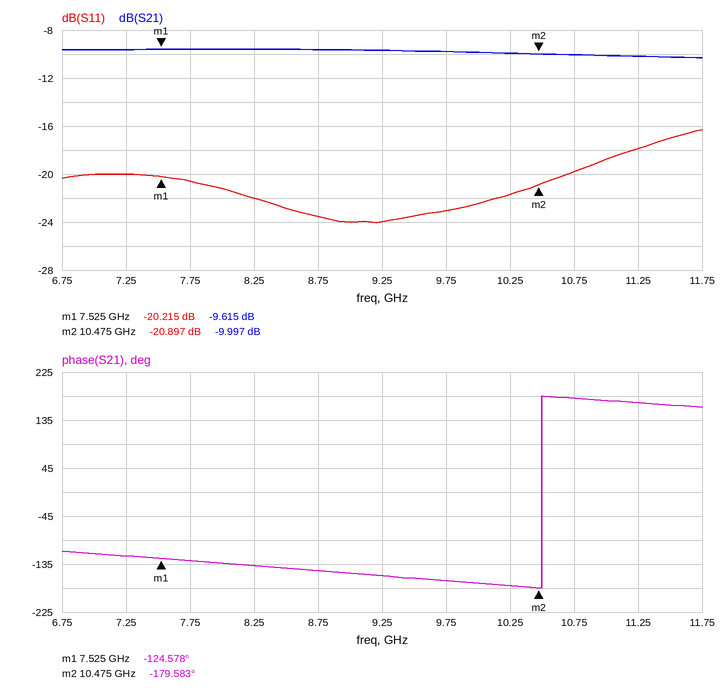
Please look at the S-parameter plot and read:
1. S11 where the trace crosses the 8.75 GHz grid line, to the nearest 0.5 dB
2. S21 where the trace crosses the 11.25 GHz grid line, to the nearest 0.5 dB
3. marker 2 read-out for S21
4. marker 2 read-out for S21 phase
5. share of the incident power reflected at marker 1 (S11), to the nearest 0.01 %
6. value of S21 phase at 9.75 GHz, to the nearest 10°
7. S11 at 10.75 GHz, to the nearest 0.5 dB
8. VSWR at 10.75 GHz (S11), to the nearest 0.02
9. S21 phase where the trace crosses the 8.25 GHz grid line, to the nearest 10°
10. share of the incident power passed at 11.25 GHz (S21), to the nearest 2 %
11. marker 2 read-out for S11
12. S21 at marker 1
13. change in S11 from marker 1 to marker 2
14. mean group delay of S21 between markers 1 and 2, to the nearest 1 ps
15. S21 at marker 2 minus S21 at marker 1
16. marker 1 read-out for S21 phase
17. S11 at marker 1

-23.5 dB
-10.0 dB
-9.997 dB
-179.583°
0.95 %
-170°
-20.0 dB
1.22
-140°
10 %
-20.897 dB
-9.615 dB
-0.682 dB
52 ps
-0.382 dB
-124.578°
-20.215 dB
